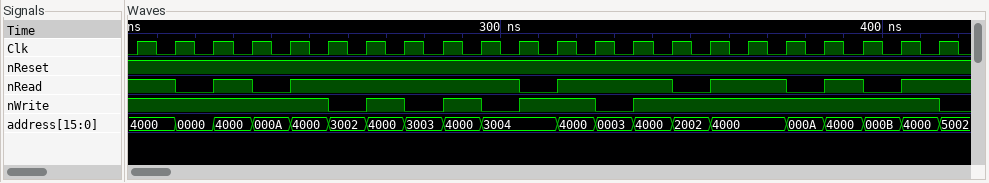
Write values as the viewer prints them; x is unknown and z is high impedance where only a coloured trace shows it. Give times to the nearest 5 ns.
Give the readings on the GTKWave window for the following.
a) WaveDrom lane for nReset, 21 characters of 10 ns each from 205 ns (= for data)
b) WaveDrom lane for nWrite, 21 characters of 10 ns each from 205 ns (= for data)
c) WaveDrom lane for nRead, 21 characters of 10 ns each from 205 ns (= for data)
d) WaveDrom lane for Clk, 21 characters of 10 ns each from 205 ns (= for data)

{name: 'nReset', wave: '1....................'}
{name: 'nWrite', wave: '1....010101.01.......'}
{name: 'nRead', wave: '10101.....01..01.0101'}
{name: 'Clk', wave: 'p....................'}
